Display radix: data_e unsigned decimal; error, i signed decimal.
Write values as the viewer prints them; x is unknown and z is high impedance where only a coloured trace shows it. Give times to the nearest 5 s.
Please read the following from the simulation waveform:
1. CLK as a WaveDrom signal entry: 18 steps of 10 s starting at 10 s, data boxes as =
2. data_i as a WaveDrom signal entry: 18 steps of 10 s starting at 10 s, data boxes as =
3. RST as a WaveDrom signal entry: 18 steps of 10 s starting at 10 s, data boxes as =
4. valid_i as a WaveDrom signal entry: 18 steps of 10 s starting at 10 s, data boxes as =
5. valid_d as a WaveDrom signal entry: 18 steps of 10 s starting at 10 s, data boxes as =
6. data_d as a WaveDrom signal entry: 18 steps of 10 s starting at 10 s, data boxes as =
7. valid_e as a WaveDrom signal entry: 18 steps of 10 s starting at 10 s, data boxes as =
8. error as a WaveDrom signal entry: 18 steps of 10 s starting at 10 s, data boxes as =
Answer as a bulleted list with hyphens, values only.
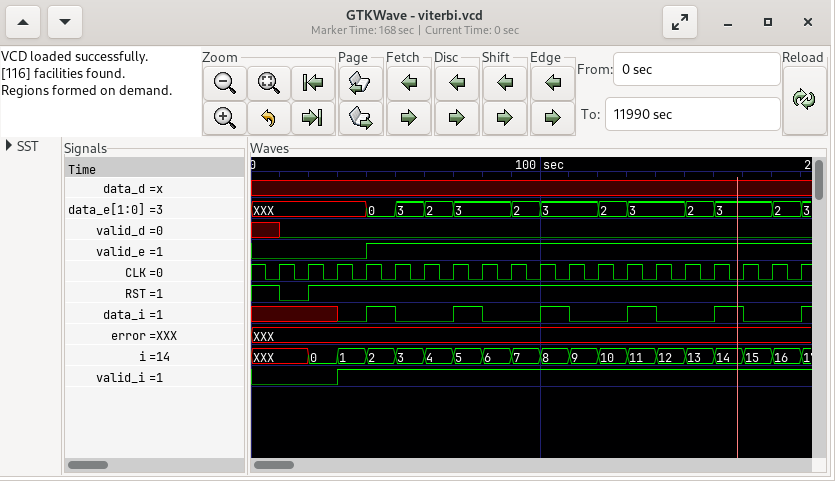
- {name: 'CLK', wave: 'p.................'}
- {name: 'data_i', wave: 'x.010.10.10.10.10.'}
- {name: 'RST', wave: '01................'}
- {name: 'valid_i', wave: '0.1...............'}
- {name: 'valid_d', wave: '0.................'}
- {name: 'data_d', wave: 'x.................'}
- {name: 'valid_e', wave: '0..1..............'}
- {name: 'error', wave: 'x.................'}
